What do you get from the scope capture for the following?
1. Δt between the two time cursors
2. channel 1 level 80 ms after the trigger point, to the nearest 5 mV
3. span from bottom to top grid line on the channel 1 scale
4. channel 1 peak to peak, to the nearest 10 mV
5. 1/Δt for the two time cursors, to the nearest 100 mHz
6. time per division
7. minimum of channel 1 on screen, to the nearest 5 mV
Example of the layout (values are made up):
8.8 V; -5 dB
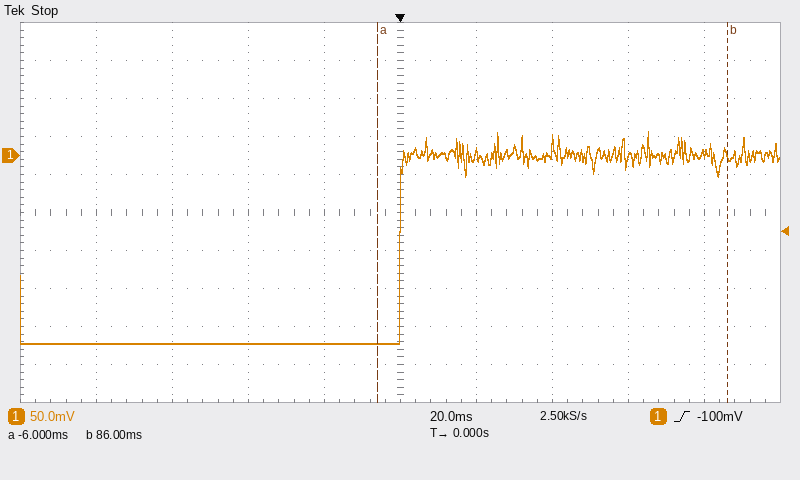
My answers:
92 ms; 5 mV; 500 mV; 280 mV; 10.9 Hz; 20 ms; -250 mV
